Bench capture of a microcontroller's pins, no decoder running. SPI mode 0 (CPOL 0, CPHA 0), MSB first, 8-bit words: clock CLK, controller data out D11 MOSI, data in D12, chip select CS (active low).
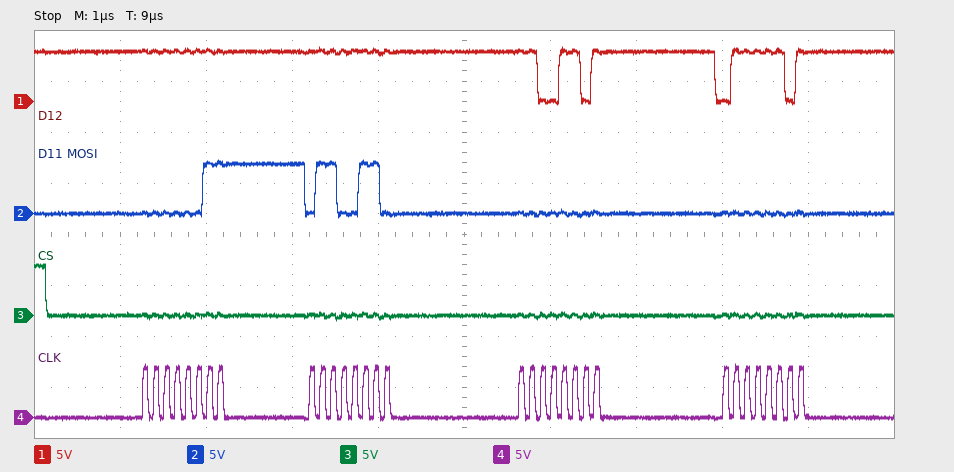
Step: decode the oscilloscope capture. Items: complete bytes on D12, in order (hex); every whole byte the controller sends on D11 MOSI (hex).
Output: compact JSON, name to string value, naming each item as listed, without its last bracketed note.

{"complete bytes on D12, in order": "FF FF CD 7D", "every whole byte the controller sends on D11 MOSI": "03 66 00 00"}
